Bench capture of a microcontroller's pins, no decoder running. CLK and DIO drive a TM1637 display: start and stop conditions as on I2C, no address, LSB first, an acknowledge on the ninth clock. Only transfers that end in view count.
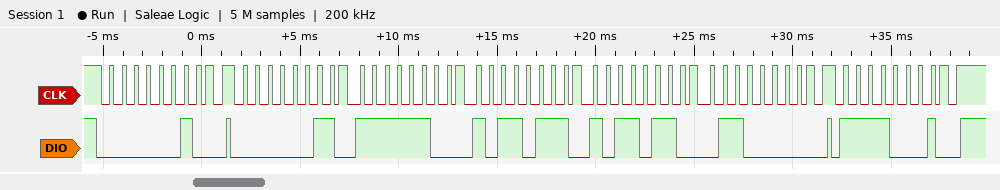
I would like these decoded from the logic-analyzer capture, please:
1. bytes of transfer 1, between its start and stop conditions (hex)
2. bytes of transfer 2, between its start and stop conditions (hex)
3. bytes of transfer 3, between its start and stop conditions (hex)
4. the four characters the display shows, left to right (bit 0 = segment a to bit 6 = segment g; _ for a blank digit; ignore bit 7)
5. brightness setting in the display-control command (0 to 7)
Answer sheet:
40
C0 3F ED 6D 06
8F
0551
7
